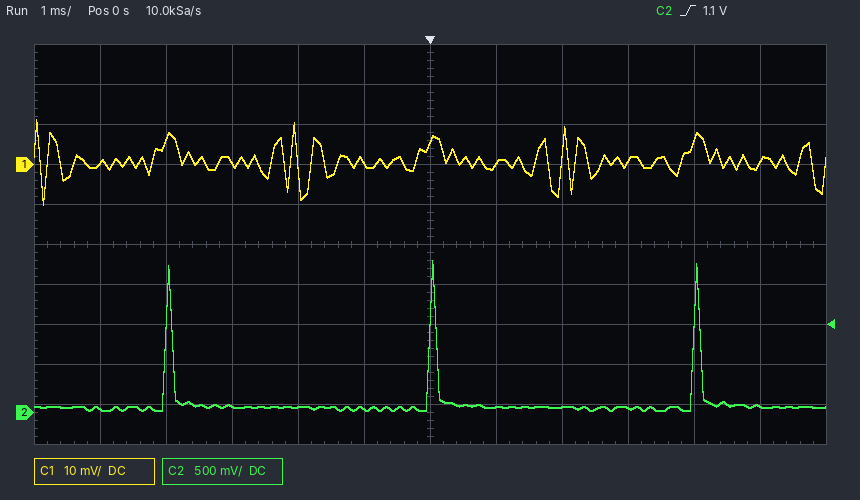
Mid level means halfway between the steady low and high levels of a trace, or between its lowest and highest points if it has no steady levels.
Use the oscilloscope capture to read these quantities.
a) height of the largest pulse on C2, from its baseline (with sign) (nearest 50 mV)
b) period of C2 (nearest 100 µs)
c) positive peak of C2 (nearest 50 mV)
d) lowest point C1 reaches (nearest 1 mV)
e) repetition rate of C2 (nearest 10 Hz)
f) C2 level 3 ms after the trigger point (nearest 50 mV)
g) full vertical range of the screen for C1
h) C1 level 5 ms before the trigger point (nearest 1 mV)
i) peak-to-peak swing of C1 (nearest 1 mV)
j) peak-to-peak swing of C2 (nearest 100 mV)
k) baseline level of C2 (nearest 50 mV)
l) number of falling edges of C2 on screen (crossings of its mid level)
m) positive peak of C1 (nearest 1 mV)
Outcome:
+1.85 V
4.0 ms
1.90 V
-10 mV
250 Hz
50 mV
100 mV
0 mV
21 mV
1.90 V
50 mV
3
11 mV
